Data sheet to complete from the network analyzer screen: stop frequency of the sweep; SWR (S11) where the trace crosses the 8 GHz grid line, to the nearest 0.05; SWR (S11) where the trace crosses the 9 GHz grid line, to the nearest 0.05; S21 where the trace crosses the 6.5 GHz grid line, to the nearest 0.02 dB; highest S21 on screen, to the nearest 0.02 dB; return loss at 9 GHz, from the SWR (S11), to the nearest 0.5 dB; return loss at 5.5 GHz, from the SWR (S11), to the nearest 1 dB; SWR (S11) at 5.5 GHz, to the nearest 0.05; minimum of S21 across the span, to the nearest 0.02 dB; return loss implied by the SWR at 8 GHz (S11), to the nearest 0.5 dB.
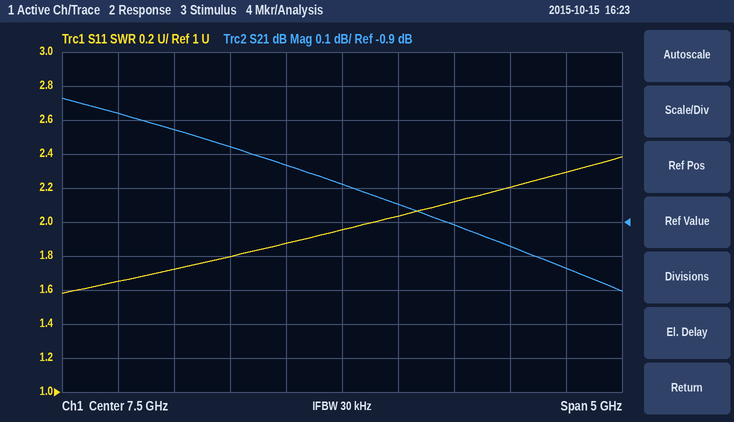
10 GHz
2.05
2.20
-0.68 dB
-0.54 dB
8.5 dB
12 dB
1.65
-1.10 dB
9.5 dB
